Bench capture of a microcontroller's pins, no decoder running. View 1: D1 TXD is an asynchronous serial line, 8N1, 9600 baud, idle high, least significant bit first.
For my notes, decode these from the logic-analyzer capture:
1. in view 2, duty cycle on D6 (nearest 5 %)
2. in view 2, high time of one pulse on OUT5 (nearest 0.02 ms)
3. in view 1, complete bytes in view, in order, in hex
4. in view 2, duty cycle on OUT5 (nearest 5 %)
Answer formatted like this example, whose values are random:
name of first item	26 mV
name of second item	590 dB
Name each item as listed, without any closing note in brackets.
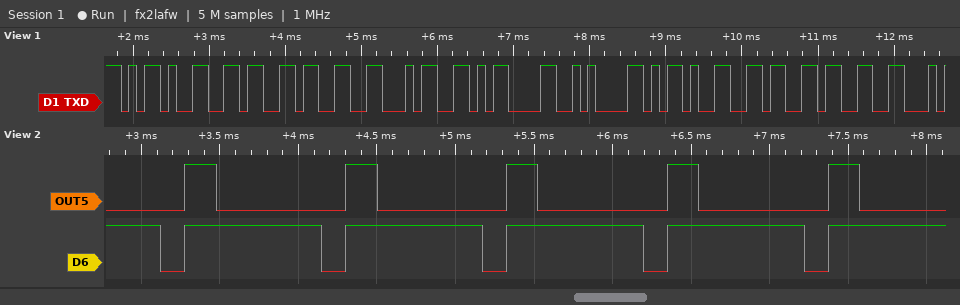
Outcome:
in view 2, duty cycle on D6	85 %
in view 2, high time of one pulse on OUT5	0.20 ms
in view 1, complete bytes in view, in order, in hex	2D 36 33 34 0D 0A 2D 36 33
in view 2, duty cycle on OUT5	20 %
